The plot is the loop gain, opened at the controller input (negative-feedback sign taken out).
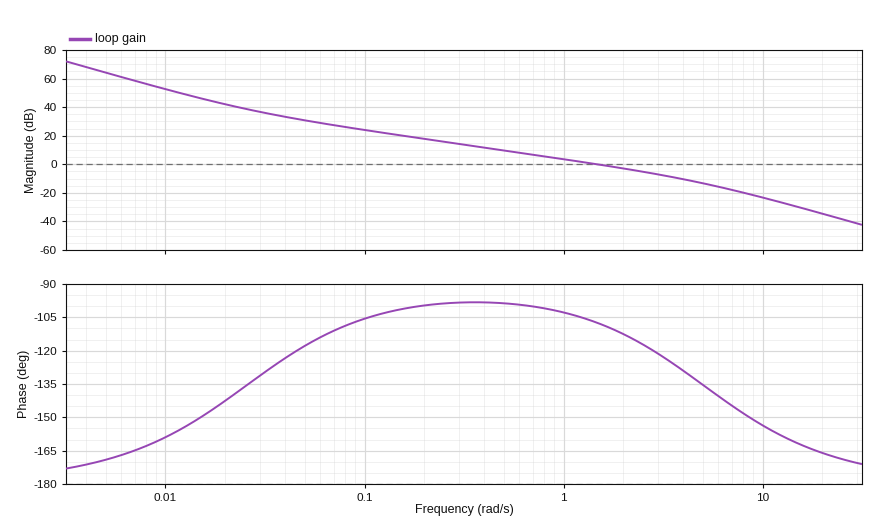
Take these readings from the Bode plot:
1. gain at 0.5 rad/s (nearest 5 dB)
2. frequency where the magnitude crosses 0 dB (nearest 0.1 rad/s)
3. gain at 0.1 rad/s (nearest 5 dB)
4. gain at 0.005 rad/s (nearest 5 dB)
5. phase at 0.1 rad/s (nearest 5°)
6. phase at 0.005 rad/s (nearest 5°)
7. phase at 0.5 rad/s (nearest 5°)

10 dB
1.5 rad/s
25 dB
65 dB
-105°
-170°
-100°
